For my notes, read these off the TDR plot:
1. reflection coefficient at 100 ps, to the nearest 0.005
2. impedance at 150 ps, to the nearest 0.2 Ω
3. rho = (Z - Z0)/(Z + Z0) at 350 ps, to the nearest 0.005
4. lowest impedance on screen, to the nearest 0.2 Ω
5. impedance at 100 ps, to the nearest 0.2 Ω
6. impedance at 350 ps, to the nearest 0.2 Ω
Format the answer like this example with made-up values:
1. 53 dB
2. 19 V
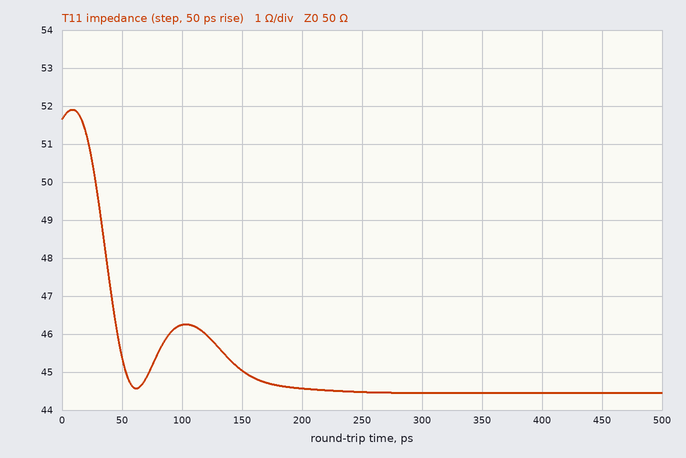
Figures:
1. -0.040
2. 45.0 Ω
3. -0.060
4. 44.4 Ω
5. 46.2 Ω
6. 44.4 Ω
